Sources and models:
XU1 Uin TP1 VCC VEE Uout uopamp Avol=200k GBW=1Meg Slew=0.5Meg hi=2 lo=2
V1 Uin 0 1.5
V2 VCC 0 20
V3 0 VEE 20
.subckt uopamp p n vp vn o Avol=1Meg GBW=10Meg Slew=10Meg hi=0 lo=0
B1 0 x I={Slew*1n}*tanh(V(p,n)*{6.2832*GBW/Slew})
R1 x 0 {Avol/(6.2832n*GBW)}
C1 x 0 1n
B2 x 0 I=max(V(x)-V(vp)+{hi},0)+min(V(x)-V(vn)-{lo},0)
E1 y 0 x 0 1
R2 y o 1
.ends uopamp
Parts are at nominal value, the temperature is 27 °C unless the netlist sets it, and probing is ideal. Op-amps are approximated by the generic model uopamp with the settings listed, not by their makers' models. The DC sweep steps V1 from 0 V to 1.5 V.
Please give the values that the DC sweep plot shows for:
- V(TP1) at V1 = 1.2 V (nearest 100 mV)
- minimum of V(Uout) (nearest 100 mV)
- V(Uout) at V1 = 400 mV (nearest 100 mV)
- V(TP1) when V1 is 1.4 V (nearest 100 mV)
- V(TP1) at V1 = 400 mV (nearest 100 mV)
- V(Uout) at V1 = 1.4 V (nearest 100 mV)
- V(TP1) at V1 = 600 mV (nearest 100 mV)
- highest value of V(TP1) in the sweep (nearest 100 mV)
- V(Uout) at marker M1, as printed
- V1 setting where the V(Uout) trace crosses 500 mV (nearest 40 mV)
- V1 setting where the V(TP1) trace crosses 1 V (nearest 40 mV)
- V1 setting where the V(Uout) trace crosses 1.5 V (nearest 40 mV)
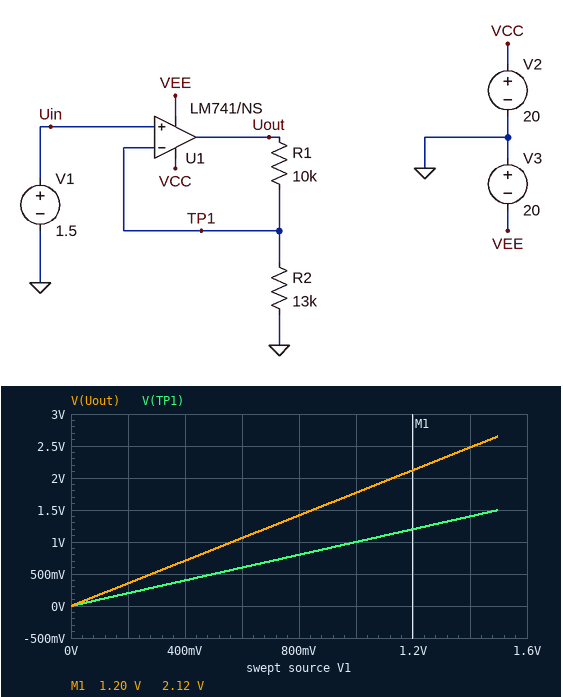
1.2 V
0 V
700 mV
1.4 V
400 mV
2.5 V
600 mV
1.5 V
2.12 V
280 mV
1.00 V
840 mV
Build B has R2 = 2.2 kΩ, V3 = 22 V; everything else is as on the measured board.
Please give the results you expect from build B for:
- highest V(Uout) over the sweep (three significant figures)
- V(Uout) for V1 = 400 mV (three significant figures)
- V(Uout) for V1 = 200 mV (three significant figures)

8.32 V
2.22 V
1.11 V
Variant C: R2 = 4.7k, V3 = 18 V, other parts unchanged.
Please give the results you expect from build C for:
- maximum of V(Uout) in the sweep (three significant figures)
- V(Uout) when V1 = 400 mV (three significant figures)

4.69 V
1.25 V
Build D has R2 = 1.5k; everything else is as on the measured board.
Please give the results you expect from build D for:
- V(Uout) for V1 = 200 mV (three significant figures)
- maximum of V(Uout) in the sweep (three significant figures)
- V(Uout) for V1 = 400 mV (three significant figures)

1.53 V
11.5 V
3.07 V
